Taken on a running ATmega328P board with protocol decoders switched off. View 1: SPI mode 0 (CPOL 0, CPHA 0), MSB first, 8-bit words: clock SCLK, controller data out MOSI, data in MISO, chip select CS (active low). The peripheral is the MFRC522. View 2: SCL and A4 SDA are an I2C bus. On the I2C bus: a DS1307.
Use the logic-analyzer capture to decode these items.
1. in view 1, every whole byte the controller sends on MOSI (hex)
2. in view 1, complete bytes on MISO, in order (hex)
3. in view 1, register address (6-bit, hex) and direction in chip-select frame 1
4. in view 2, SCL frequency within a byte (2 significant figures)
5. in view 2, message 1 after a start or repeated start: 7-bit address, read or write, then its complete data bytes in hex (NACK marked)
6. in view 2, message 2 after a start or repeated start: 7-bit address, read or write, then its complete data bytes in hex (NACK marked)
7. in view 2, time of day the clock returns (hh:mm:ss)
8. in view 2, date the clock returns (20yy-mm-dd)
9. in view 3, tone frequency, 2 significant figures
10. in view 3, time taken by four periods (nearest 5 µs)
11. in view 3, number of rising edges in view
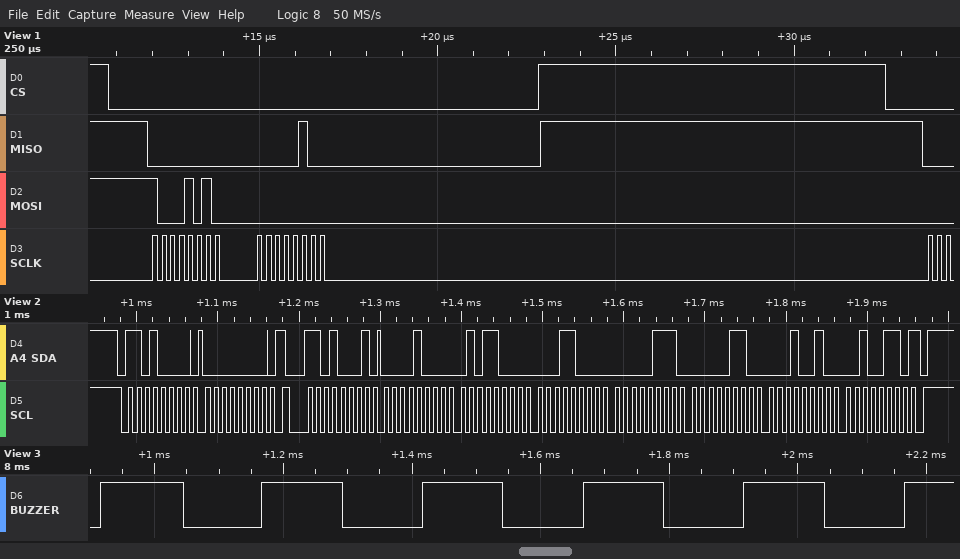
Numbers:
8A 00
00 04
0x05 read
100 kHz
0x68 write: 00
0x68 read: 08 58 18 07 06 12 26 NACK
18:58:08
2026-12-06
4.0 kHz
1000 µs
6
